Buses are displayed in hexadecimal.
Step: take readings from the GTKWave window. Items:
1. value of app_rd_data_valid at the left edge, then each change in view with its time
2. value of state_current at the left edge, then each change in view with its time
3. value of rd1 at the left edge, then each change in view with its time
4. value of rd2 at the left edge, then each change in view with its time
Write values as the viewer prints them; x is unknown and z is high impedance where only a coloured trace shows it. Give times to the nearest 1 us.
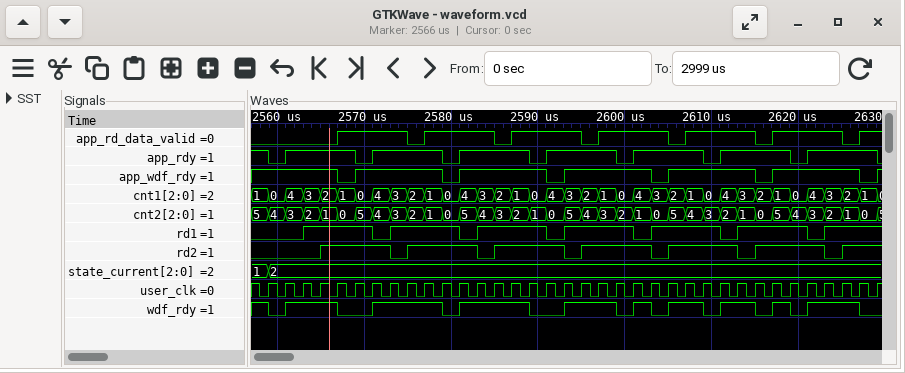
0, 1 at 2567 us, 0 at 2575 us, 1 at 2577 us, 0 at 2585 us, 1 at 2587 us, 0 at 2595 us, 1 at 2597 us, 0 at 2605 us, 1 at 2607 us, 0 at 2615 us, 1 at 2617 us, 0 at 2625 us, 1 at 2627 us
1, 2 at 2559 us
0, 1 at 2563 us, 0 at 2571 us, 1 at 2573 us, 0 at 2581 us, 1 at 2583 us, 0 at 2591 us, 1 at 2593 us, 0 at 2601 us, 1 at 2603 us, 0 at 2611 us, 1 at 2613 us, 0 at 2621 us, 1 at 2623 us
0, 1 at 2565 us, 0 at 2573 us, 1 at 2575 us, 0 at 2583 us, 1 at 2585 us, 0 at 2593 us, 1 at 2595 us, 0 at 2603 us, 1 at 2605 us, 0 at 2613 us, 1 at 2615 us, 0 at 2623 us, 1 at 2625 us
